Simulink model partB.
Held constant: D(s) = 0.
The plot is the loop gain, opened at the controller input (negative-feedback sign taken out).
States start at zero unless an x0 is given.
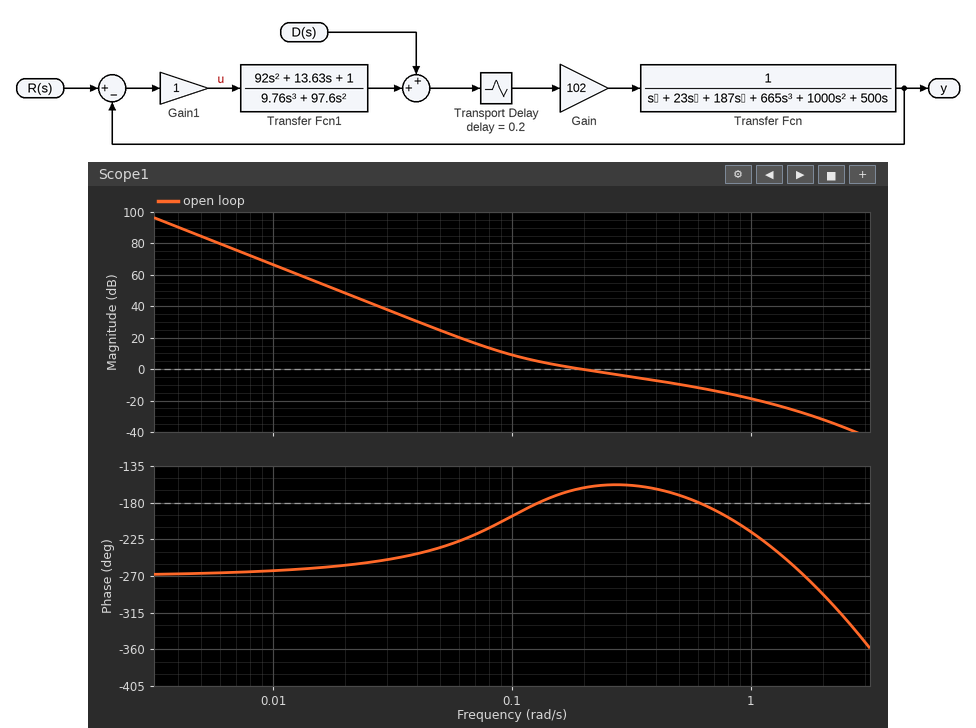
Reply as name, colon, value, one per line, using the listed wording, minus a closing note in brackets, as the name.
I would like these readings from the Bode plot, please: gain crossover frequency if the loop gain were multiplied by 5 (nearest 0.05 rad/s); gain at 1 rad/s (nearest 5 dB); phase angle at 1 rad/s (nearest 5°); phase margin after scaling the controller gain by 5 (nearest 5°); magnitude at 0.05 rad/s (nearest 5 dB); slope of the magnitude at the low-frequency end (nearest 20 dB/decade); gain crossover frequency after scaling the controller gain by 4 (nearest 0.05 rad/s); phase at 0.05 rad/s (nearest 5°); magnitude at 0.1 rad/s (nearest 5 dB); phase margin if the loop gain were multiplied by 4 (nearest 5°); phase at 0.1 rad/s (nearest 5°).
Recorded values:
gain crossover frequency if the loop gain were multiplied by 5: 0.70 rad/s
gain at 1 rad/s: -20 dB
phase angle at 1 rad/s: -215°
phase margin after scaling the controller gain by 5: -10°
magnitude at 0.05 rad/s: 25 dB
slope of the magnitude at the low-frequency end: -60 dB/decade
gain crossover frequency after scaling the controller gain by 4: 0.60 rad/s
phase at 0.05 rad/s: -235°
magnitude at 0.1 rad/s: 10 dB
phase margin if the loop gain were multiplied by 4: 0°
phase at 0.1 rad/s: -195°
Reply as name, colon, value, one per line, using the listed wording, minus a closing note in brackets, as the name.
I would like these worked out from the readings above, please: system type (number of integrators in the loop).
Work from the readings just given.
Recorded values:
system type: 3
